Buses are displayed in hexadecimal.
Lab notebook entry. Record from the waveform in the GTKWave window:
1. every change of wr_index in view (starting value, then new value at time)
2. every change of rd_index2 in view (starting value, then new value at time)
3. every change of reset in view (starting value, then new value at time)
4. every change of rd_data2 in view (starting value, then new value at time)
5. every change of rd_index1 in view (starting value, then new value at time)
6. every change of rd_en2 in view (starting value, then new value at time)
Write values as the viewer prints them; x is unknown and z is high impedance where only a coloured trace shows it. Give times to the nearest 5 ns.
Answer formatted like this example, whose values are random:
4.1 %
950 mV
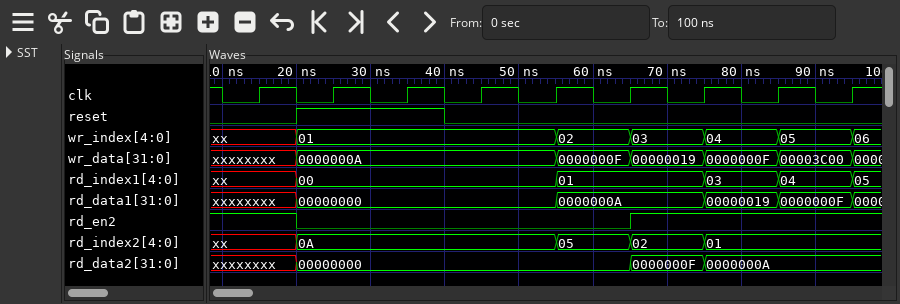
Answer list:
xx, 01 at 20 ns, 02 at 55 ns, 03 at 65 ns, 04 at 75 ns, 05 at 85 ns, 06 at 95 ns
xx, 0A at 20 ns, 05 at 55 ns, 02 at 65 ns, 01 at 75 ns
0, 1 at 20 ns, 0 at 40 ns
xxxxxxxx, 00000000 at 20 ns, 0000000F at 65 ns, 0000000A at 75 ns
xx, 00 at 20 ns, 01 at 55 ns, 03 at 75 ns, 04 at 85 ns, 05 at 95 ns
1, 0 at 20 ns, 1 at 65 ns
